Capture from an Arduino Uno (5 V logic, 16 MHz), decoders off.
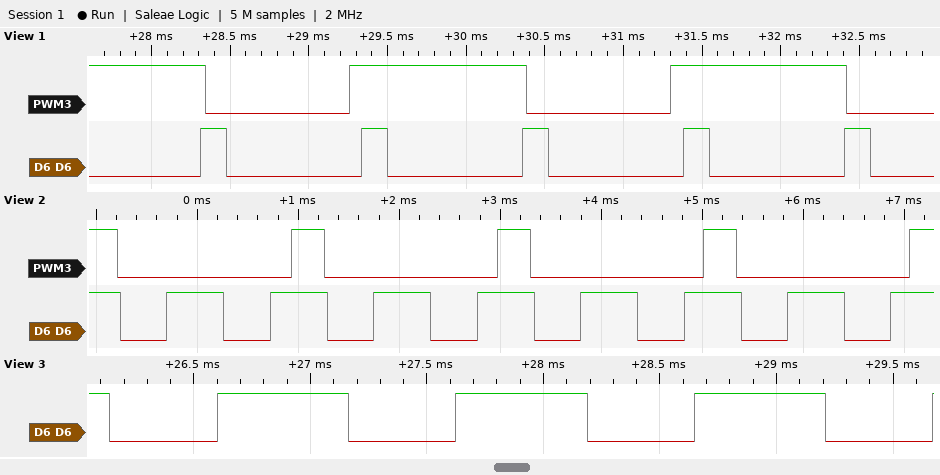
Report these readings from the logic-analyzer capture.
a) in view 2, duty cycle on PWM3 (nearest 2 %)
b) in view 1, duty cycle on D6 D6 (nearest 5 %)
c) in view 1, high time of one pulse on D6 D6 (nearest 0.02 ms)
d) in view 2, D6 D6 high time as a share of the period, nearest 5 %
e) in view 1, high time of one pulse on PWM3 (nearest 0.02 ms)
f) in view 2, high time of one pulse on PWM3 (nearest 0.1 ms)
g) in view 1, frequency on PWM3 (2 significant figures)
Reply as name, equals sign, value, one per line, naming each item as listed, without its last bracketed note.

in view 2, duty cycle on PWM3 = 16 %
in view 1, duty cycle on D6 D6 = 15 %
in view 1, high time of one pulse on D6 D6 = 0.16 ms
in view 2, D6 D6 high time as a share of the period, nearest 5 % = 55 %
in view 1, high time of one pulse on PWM3 = 1.12 ms
in view 2, high time of one pulse on PWM3 = 0.3 ms
in view 1, frequency on PWM3 = 490 Hz
